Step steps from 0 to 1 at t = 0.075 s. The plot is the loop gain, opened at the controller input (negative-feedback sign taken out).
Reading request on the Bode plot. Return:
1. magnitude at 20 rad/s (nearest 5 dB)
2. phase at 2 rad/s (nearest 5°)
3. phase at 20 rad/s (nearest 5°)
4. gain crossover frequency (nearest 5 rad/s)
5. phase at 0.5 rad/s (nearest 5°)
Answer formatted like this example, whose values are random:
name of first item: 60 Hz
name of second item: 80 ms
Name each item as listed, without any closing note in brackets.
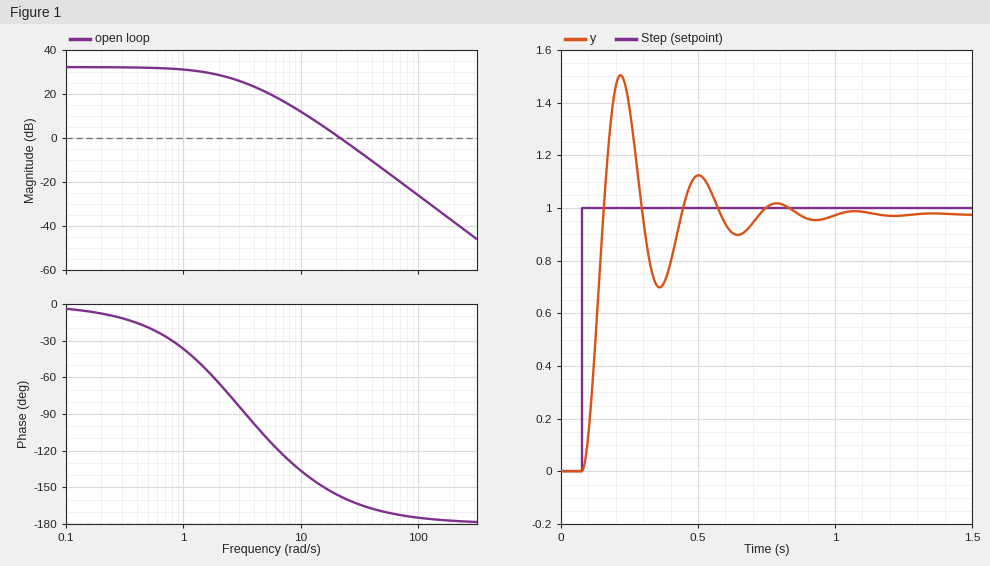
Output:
magnitude at 20 rad/s: 0 dB
phase at 2 rad/s: -65°
phase at 20 rad/s: -155°
gain crossover frequency: 20 rad/s
phase at 0.5 rad/s: -20°
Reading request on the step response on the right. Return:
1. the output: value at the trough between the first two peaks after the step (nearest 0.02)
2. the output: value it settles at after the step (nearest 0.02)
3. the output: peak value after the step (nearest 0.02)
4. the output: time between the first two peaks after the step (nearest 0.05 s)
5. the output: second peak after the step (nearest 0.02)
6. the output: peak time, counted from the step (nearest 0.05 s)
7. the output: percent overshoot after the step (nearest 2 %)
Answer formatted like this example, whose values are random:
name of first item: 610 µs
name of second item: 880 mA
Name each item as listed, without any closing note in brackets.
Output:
the output: value at the trough between the first two peaks after the step: 0.70
the output: value it settles at after the step: 0.98
the output: peak value after the step: 1.50
the output: time between the first two peaks after the step: 0.30 s
the output: second peak after the step: 1.12
the output: peak time, counted from the step: 0.15 s
the output: percent overshoot after the step: 54 %
